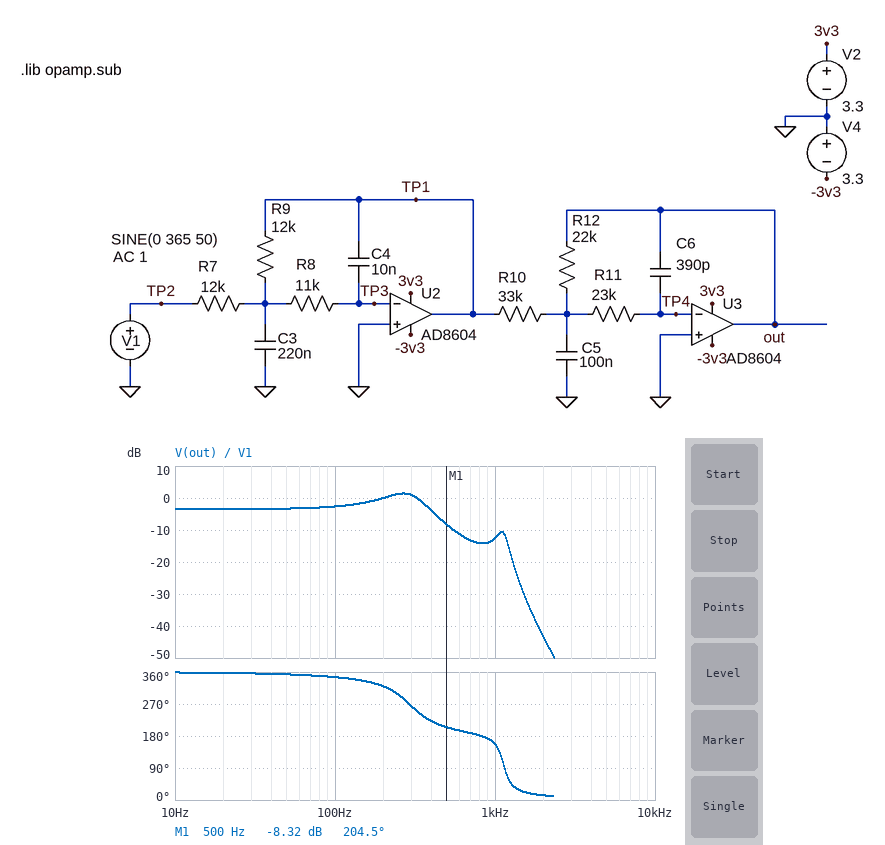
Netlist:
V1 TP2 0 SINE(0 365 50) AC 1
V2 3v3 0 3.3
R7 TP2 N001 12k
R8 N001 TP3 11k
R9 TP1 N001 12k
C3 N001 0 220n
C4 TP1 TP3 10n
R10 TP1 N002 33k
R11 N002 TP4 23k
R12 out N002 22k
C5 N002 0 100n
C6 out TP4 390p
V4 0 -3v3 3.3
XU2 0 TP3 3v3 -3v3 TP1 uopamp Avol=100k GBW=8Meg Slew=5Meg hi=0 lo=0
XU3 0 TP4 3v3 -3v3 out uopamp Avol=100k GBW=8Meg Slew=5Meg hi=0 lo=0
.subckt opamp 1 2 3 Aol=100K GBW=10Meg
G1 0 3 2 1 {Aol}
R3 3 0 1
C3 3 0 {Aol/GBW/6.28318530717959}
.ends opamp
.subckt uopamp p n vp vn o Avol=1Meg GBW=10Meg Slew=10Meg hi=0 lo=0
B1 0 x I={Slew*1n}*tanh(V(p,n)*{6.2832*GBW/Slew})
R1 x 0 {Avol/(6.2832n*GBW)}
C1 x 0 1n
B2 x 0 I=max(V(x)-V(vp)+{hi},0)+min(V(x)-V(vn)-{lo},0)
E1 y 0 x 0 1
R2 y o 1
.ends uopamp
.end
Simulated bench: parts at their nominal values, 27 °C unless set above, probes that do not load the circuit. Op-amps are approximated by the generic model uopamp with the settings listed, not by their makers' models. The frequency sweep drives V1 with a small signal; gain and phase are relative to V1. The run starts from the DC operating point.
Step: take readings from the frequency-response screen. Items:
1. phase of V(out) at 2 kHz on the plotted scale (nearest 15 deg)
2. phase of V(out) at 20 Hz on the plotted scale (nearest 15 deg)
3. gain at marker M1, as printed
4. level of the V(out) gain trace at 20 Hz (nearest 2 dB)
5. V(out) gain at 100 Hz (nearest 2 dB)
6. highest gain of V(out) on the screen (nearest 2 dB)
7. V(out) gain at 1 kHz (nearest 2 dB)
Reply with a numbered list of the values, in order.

1. 15 deg
2. 360 deg
3. -8.32 dB
4. -4 dB
5. -2 dB
6. 2 dB
7. -12 dB
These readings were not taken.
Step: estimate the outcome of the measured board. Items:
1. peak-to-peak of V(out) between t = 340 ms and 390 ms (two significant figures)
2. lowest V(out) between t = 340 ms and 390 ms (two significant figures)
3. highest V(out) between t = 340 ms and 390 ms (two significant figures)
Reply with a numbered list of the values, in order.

1. 6.6 V
2. -3.3 V
3. 3.3 V
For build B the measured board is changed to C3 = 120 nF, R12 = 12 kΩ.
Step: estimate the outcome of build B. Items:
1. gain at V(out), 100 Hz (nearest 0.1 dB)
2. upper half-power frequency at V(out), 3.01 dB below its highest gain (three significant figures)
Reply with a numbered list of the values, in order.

1. -8.4 dB
2. 490 Hz
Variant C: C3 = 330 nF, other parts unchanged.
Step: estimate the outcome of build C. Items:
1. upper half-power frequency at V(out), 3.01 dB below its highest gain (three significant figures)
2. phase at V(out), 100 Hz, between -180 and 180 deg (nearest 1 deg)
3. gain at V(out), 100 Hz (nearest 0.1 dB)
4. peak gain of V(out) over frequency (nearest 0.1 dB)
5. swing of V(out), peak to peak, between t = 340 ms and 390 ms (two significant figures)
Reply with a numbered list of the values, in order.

1. 284 Hz
2. -15 deg
3. -2.1 dB
4. 2.9 dB
5. 6.6 V
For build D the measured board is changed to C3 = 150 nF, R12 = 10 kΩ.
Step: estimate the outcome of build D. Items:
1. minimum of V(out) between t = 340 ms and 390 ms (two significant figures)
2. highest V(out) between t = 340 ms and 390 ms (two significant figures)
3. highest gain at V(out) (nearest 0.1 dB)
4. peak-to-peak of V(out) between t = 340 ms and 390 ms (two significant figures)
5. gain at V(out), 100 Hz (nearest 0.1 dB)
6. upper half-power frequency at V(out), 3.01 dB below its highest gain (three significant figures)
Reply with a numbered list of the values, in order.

1. -2.5 V
2. 2.5 V
3. -7.1 dB
4. 5.0 V
5. -9.9 dB
6. 433 Hz
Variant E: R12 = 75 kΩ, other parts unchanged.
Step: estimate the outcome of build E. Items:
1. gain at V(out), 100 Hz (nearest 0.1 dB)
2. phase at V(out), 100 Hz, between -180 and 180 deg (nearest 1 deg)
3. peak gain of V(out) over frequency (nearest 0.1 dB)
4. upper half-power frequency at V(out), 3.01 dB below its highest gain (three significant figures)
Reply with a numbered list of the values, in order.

1. 8.2 dB
2. -16 deg
3. 13.4 dB
4. 390 Hz
